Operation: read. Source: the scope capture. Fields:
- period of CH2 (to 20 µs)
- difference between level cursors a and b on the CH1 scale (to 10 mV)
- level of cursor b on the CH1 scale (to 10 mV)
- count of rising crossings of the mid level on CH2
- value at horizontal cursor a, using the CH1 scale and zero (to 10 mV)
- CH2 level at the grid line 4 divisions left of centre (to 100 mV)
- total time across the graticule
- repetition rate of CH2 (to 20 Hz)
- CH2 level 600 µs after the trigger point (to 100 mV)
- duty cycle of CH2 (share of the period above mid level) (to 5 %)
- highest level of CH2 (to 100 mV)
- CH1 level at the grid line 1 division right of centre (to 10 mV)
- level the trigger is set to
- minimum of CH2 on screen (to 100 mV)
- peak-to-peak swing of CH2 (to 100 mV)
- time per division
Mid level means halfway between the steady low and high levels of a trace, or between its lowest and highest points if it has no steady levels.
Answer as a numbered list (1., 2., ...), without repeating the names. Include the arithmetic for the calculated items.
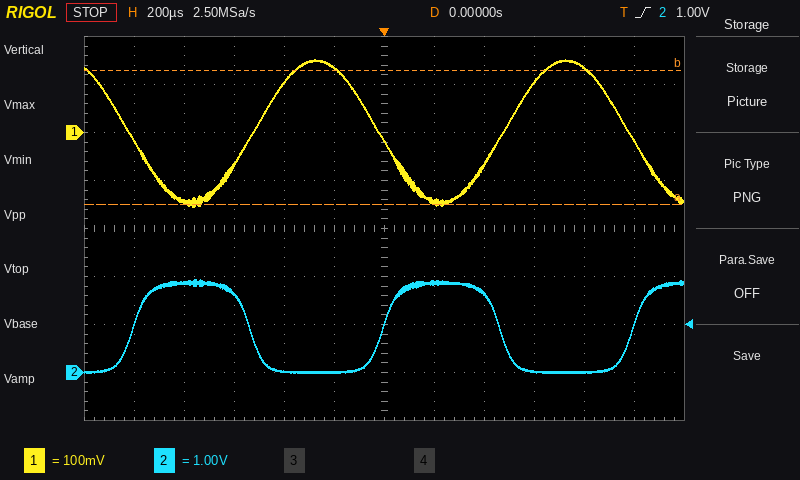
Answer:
1. 1.00 ms
2. 280 mV
3. 130 mV
4. 3
5. -150 mV
6. 1.9 V
7. 2.4 ms
8. 1 / 1.00 ms ≈ 1.00 kHz
9. 0.0 V
10. 45 %
11. 1.9 V
12. -140 mV
13. 1.00 V
14. 0.0 V
15. 1.9 V − (0.0 V) = 1.9 V
16. 200 µs
